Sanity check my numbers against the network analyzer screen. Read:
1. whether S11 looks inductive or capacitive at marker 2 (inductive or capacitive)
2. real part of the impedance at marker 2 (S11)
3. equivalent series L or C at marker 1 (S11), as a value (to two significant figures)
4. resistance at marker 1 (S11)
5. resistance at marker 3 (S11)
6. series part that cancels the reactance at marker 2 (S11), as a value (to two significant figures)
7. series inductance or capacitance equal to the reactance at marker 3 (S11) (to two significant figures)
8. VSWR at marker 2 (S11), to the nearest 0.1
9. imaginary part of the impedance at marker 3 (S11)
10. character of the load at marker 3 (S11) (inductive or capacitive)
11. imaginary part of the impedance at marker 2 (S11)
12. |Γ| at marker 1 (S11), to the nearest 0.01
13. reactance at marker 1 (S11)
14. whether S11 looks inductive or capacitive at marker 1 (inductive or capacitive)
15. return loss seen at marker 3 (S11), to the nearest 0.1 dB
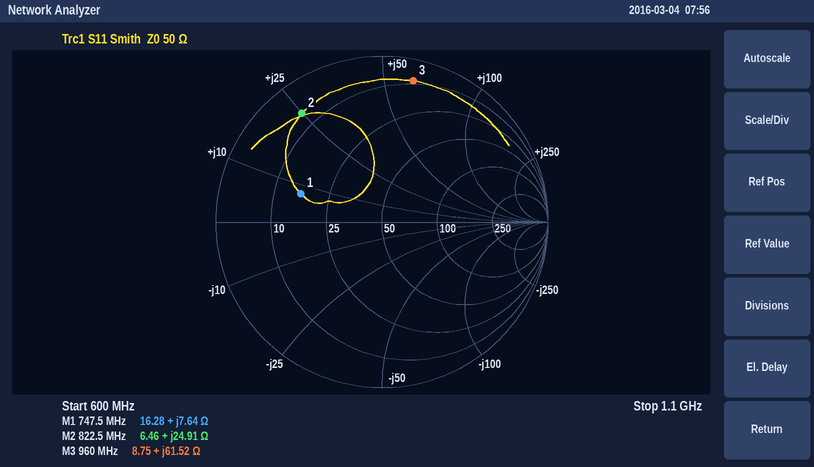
inductive
6.46 Ω
1.6 nH
16.28 Ω
8.75 Ω
7.8 pF
10 nH
9.7
+61.52 Ω
inductive
+24.91 Ω
0.52
+7.64 Ω
inductive
1.2 dB
